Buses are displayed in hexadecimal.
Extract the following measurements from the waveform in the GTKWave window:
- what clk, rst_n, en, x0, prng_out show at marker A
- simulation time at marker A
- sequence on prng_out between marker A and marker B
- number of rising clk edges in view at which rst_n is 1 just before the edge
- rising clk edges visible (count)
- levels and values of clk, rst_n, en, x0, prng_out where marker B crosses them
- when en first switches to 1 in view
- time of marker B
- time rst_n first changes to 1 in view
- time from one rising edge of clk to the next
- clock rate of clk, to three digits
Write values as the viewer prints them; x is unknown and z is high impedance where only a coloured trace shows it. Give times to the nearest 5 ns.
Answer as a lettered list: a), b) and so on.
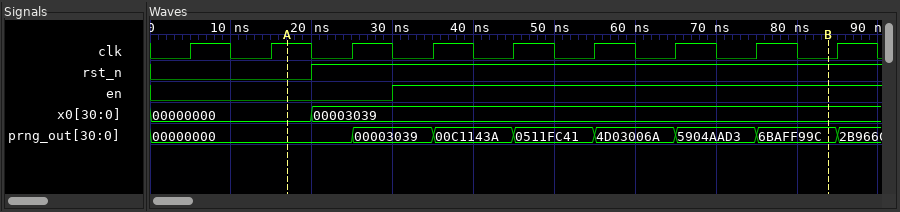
a) clk=1, rst_n=0, en=0, x0=00000000, prng_out=00000000
b) 15 ns
c) 00000000, 00003039, 00C1143A, 0511FC41, 4D03006A, 5904AAD3, 6BAFF99C
d) 7
e) 9
f) clk=0, rst_n=1, en=1, x0=00003039, prng_out=6BAFF99C
g) 30 ns
h) 85 ns
i) 20 ns
j) 10 ns
k) 100 MHz
